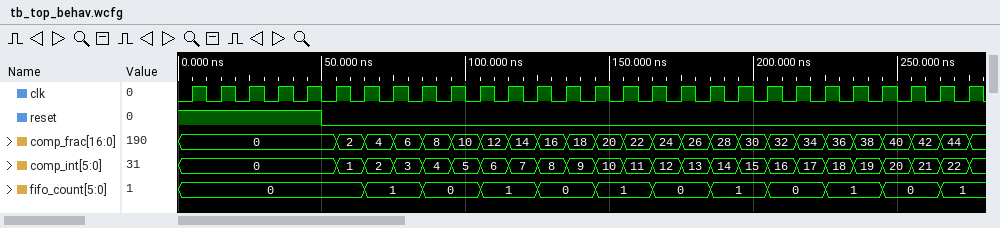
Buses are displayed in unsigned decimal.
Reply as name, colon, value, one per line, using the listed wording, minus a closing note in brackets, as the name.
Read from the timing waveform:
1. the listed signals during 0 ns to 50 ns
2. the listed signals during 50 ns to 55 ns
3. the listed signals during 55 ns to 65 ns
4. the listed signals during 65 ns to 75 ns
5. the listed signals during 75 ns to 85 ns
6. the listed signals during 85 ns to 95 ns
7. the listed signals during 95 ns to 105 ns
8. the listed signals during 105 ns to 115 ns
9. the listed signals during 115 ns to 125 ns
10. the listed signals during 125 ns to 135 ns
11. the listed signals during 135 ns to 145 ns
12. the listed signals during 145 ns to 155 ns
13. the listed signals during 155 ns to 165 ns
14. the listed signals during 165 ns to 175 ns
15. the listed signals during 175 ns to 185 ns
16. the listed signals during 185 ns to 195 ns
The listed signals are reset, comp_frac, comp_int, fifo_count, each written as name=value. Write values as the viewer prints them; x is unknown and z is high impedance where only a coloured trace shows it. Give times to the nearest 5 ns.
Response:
the listed signals during 0 ns to 50 ns: reset=1, comp_frac=0, comp_int=0, fifo_count=0
the listed signals during 50 ns to 55 ns: reset=0, comp_frac=0, comp_int=0, fifo_count=0
the listed signals during 55 ns to 65 ns: reset=0, comp_frac=2, comp_int=1, fifo_count=0
the listed signals during 65 ns to 75 ns: reset=0, comp_frac=4, comp_int=2, fifo_count=1
the listed signals during 75 ns to 85 ns: reset=0, comp_frac=6, comp_int=3, fifo_count=1
the listed signals during 85 ns to 95 ns: reset=0, comp_frac=8, comp_int=4, fifo_count=0
the listed signals during 95 ns to 105 ns: reset=0, comp_frac=10, comp_int=5, fifo_count=0
the listed signals during 105 ns to 115 ns: reset=0, comp_frac=12, comp_int=6, fifo_count=1
the listed signals during 115 ns to 125 ns: reset=0, comp_frac=14, comp_int=7, fifo_count=1
the listed signals during 125 ns to 135 ns: reset=0, comp_frac=16, comp_int=8, fifo_count=0
the listed signals during 135 ns to 145 ns: reset=0, comp_frac=18, comp_int=9, fifo_count=0
the listed signals during 145 ns to 155 ns: reset=0, comp_frac=20, comp_int=10, fifo_count=1
the listed signals during 155 ns to 165 ns: reset=0, comp_frac=22, comp_int=11, fifo_count=1
the listed signals during 165 ns to 175 ns: reset=0, comp_frac=24, comp_int=12, fifo_count=0
the listed signals during 175 ns to 185 ns: reset=0, comp_frac=26, comp_int=13, fifo_count=0
the listed signals during 185 ns to 195 ns: reset=0, comp_frac=28, comp_int=14, fifo_count=1
